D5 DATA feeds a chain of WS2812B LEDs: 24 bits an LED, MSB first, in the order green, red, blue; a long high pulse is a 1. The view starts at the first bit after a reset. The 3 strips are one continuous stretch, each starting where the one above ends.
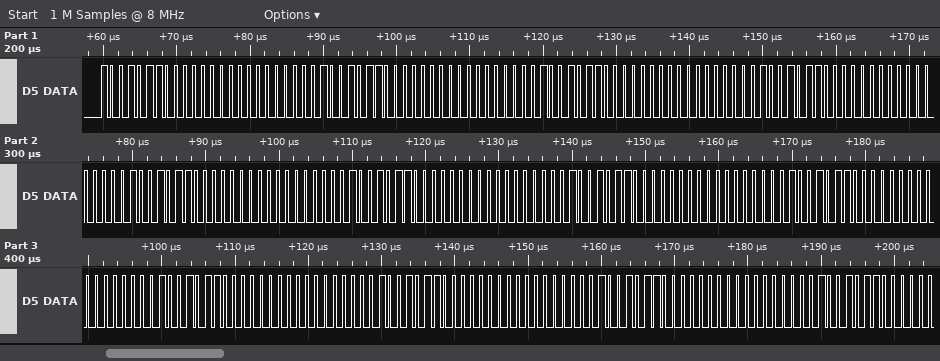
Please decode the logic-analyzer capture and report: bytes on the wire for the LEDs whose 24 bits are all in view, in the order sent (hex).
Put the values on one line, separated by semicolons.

96 00 00 96 00 00 96 00 00 96 00 00 96 00 00 96 00 00 96 00 00 96 00 00 96 00 00 96 00 00 96 00 00
